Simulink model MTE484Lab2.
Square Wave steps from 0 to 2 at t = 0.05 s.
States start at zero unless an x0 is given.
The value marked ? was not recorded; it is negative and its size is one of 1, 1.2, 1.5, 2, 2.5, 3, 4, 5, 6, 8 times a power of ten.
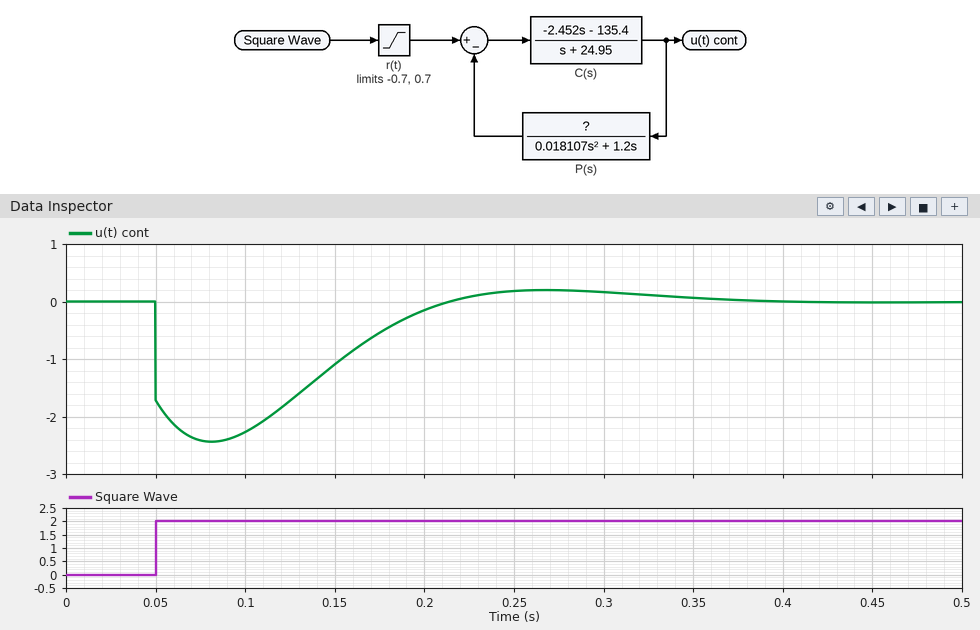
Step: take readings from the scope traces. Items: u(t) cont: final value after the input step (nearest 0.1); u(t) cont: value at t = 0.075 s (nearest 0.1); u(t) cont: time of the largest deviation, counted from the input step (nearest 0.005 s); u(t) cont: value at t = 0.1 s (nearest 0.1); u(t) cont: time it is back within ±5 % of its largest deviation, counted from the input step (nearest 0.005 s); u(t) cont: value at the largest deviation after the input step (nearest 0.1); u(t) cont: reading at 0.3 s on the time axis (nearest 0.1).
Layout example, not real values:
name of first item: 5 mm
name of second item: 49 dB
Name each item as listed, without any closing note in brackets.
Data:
u(t) cont: final value after the input step: 0.0
u(t) cont: value at t = 0.075 s: -2.4
u(t) cont: time of the largest deviation, counted from the input step: 0.030 s
u(t) cont: value at t = 0.1 s: -2.3
u(t) cont: time it is back within ±5 % of its largest deviation, counted from the input step: 0.270 s
u(t) cont: value at the largest deviation after the input step: -2.4
u(t) cont: reading at 0.3 s on the time axis: 0.2
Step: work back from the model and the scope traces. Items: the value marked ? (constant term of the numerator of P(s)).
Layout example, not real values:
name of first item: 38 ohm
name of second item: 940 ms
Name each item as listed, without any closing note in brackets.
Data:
the value marked ? (constant term of the numerator of P(s)): -4
